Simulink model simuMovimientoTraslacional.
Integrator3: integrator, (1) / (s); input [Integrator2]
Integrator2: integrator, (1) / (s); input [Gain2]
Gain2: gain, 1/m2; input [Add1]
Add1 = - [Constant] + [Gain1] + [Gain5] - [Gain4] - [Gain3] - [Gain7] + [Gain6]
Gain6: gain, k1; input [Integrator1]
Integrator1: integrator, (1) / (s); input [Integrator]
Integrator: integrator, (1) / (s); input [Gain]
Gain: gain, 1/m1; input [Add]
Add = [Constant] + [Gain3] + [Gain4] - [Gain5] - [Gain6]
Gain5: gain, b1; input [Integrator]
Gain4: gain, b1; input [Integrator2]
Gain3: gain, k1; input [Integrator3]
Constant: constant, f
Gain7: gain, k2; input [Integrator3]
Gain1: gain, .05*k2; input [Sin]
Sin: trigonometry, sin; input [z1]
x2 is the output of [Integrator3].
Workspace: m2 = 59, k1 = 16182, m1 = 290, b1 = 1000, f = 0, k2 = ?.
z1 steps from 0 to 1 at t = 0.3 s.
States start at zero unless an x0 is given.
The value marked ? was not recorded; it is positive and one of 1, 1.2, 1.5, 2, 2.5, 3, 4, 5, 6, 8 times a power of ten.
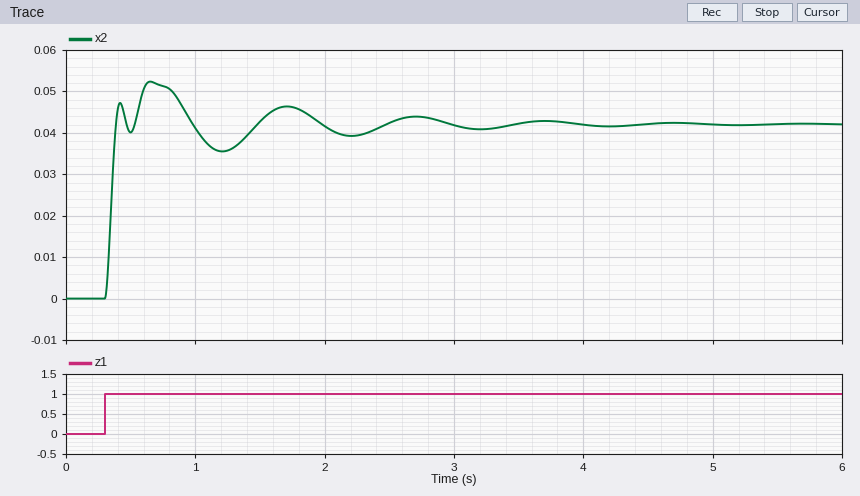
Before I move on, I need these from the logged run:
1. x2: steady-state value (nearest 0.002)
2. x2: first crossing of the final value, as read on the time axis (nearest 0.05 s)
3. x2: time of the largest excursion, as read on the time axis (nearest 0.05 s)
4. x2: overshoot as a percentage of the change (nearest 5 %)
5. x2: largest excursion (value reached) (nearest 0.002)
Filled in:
0.042
0.40 s
0.65 s
25 %
0.052
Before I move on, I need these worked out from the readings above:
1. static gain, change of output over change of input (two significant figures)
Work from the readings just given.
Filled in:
0.042
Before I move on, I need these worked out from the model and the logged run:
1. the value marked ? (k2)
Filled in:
40000
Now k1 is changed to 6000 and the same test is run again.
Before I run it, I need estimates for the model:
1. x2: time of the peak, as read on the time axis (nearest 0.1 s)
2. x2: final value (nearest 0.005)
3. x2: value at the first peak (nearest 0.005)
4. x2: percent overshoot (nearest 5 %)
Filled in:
0.4 s
0.040
0.055
30 %
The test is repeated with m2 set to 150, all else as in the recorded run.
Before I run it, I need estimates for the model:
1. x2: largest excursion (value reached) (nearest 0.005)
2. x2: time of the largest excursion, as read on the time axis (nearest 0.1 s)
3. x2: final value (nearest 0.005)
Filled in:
0.055
0.8 s
0.040
